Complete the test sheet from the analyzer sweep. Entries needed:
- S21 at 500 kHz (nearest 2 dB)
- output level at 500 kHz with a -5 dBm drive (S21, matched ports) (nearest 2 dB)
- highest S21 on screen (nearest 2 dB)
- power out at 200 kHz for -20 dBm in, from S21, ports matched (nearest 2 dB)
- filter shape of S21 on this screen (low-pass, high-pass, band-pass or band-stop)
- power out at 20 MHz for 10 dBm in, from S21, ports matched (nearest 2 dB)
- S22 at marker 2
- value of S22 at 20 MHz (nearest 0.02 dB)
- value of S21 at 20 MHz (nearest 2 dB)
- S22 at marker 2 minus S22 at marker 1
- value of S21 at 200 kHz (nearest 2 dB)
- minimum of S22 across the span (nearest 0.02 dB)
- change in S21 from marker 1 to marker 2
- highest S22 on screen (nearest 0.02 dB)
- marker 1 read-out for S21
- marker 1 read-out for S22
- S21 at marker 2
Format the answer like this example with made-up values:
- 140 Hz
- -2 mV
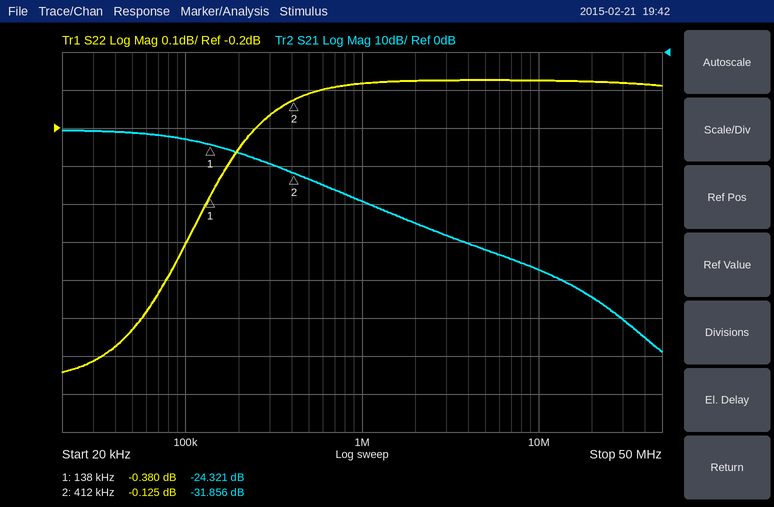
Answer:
- -34 dB
- -38 dBm
- -20 dB
- -46 dBm
- low-pass
- -54 dBm
- -0.125 dB
- -0.08 dB
- -64 dB
- 0.255 dB
- -26 dB
- -0.84 dB
- -7.535 dB
- -0.08 dB
- -24.321 dB
- -0.380 dB
- -31.856 dB
